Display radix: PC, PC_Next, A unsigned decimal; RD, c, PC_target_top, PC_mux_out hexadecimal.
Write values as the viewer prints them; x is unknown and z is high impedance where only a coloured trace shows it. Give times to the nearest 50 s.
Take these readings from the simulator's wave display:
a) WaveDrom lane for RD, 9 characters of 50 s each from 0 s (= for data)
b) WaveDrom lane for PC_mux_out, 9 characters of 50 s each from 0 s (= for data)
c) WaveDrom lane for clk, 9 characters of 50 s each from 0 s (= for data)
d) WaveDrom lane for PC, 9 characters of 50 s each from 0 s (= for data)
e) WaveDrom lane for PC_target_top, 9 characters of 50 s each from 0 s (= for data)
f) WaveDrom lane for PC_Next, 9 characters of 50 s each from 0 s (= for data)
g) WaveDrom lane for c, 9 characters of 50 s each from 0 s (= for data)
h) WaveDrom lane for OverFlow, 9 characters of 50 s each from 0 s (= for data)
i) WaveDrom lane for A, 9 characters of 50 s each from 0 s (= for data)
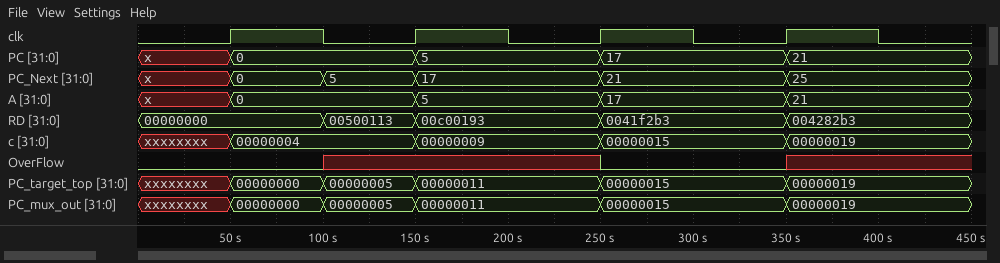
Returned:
{name: 'RD', wave: '=.==.=.=.', data: '00000000 00500113 00c00193 0041f2b3 004282b3'}
{name: 'PC_mux_out', wave: 'x===.=.=.', data: '00000000 00000005 00000011 00000015 00000019'}
{name: 'clk', wave: '010101010'}
{name: 'PC', wave: 'x=.=.=.=.', data: '0 5 17 21'}
{name: 'PC_target_top', wave: 'x===.=.=.', data: '00000000 00000005 00000011 00000015 00000019'}
{name: 'PC_Next', wave: 'x===.=.=.', data: '0 5 17 21 25'}
{name: 'c', wave: 'x=.=.=.=.', data: '00000004 00000009 00000015 00000019'}
{name: 'OverFlow', wave: '0.x..0.x.'}
{name: 'A', wave: 'x=.=.=.=.', data: '0 5 17 21'}
